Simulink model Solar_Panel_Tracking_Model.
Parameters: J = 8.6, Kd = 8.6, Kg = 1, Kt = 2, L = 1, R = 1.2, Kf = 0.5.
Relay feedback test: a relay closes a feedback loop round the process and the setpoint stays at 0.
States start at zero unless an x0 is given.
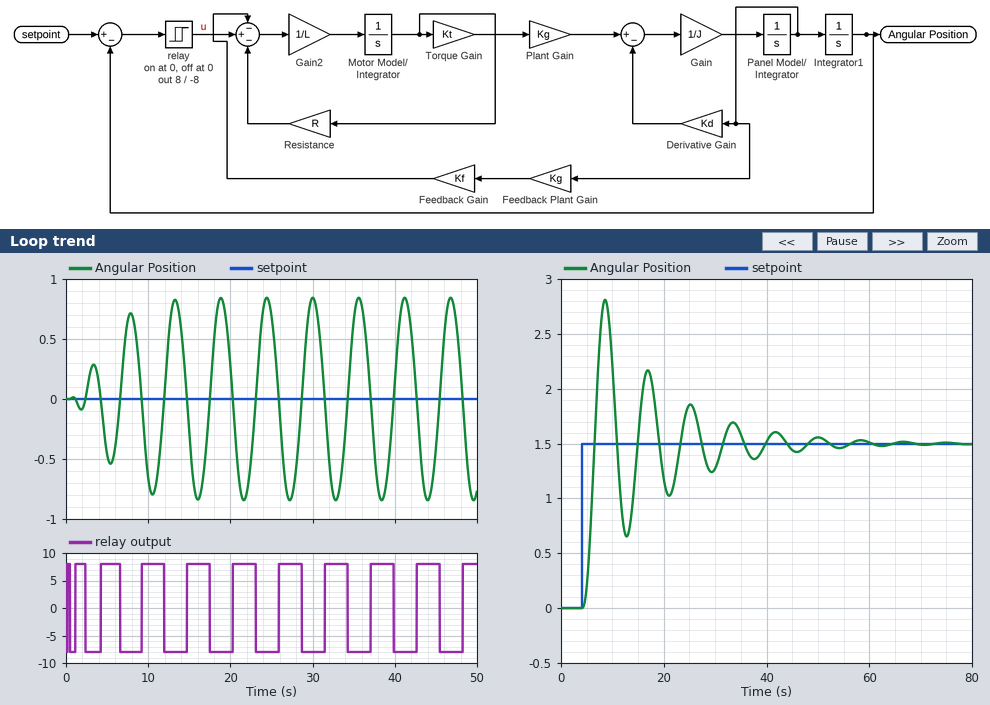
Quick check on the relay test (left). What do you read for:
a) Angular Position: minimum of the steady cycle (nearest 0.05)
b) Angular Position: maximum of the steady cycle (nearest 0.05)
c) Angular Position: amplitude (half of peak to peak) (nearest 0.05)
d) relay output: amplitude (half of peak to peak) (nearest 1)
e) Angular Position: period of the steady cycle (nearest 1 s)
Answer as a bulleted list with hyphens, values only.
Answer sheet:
- -0.85
- 0.85
- 0.85
- 8
- 6 s
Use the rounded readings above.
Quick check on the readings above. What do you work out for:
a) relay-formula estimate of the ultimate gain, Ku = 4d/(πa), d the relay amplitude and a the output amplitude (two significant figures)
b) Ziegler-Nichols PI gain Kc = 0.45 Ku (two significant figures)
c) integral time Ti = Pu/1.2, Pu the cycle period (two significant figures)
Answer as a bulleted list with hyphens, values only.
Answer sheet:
- 12
- 5.4
- 5.0 s
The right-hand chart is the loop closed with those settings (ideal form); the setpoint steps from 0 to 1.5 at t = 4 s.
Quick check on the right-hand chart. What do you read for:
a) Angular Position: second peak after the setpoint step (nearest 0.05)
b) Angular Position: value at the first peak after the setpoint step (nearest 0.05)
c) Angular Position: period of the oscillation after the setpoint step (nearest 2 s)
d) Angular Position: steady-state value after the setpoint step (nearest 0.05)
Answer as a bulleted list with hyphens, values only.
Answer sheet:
- 2.15
- 2.80
- 8 s
- 1.50
